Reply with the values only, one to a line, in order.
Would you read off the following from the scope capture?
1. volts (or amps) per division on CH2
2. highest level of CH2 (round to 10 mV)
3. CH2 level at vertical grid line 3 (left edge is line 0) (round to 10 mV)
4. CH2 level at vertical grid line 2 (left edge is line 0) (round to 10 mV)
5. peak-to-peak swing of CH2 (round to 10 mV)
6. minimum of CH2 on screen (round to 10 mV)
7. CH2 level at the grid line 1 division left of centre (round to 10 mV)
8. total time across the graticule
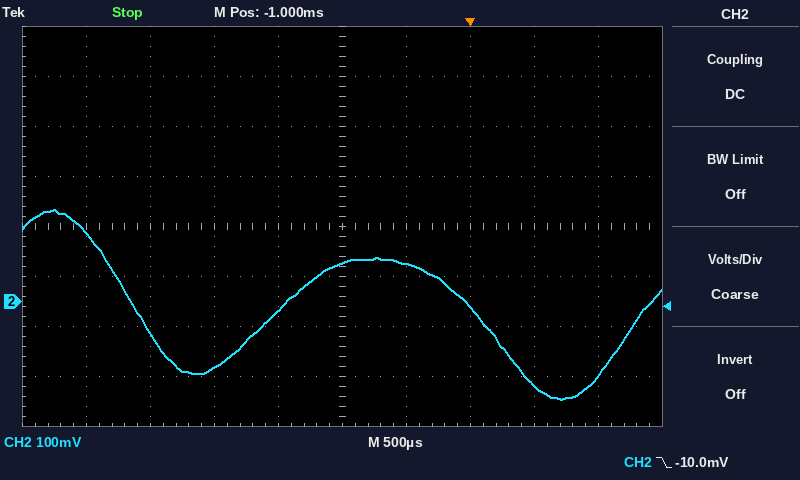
100 mV
180 mV
-130 mV
-60 mV
380 mV
-200 mV
-20 mV
5 ms
